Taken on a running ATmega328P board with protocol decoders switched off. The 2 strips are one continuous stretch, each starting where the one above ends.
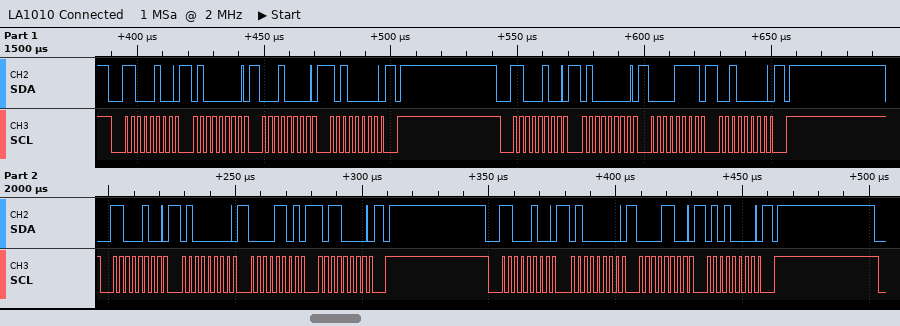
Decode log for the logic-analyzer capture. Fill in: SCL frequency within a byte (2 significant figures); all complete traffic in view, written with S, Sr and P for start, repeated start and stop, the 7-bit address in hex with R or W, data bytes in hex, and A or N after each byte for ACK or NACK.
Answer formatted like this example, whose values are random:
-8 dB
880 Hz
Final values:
400 kHz
S 62W A 40 A 10 A A0 A P S 62W A 40 A 0F A 20 A P S 62W A 40 A 0D A B0 A P S 62W A 40 A 0C A 50 A P
